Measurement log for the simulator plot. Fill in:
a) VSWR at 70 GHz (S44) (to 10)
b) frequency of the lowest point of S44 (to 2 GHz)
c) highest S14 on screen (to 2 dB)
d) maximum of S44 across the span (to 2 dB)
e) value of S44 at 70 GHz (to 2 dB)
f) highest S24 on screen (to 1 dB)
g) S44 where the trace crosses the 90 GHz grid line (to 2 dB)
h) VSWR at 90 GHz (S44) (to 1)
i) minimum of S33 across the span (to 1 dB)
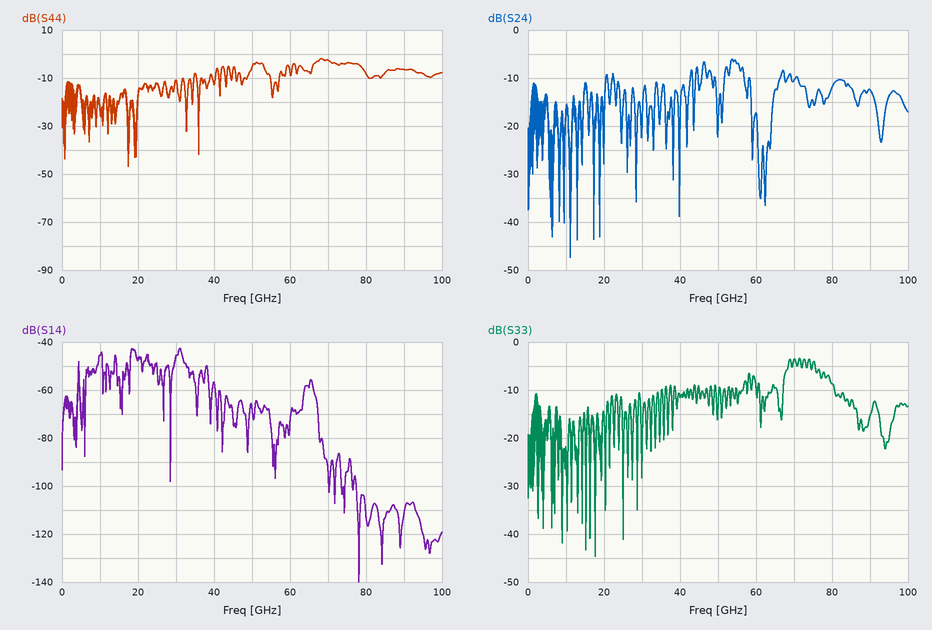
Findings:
10
18 GHz
-42 dB
-2 dB
-2 dB
-6 dB
-6 dB
3
-45 dB
